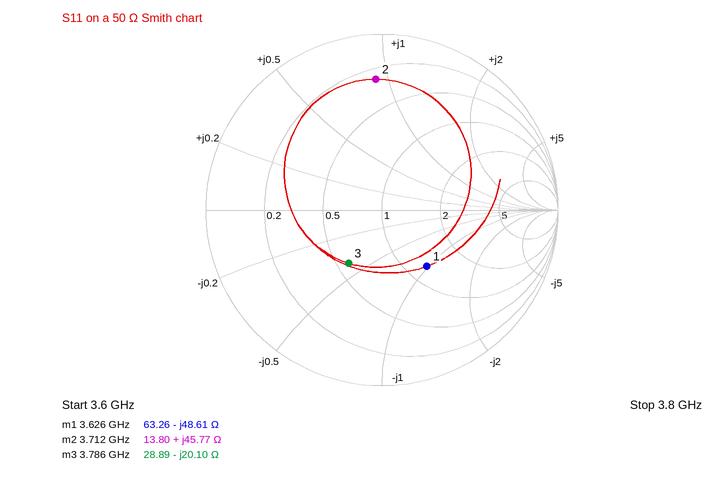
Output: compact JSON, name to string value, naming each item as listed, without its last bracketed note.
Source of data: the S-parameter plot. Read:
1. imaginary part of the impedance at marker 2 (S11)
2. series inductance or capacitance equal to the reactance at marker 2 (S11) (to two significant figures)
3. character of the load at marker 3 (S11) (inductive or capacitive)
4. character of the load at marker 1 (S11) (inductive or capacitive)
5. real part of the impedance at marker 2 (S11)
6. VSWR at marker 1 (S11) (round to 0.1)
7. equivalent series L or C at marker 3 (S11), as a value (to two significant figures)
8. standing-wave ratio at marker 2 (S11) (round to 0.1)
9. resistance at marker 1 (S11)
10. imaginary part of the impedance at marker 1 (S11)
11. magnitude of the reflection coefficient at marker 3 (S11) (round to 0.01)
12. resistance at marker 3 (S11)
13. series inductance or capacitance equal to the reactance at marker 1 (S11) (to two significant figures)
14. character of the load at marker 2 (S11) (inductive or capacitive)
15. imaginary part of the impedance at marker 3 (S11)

{"imaginary part of the impedance at marker 2": "+45.77 Ω", "series inductance or capacitance equal to the reactance at marker 2 (S11)": "2.0 nH", "character of the load at marker 3 (S11)": "capacitive", "character of the load at marker 1 (S11)": "capacitive", "real part of the impedance at marker 2": "13.80 Ω", "VSWR at marker 1 (S11)": "2.4", "equivalent series L or C at marker 3 (S11), as a value": "2.1 pF", "standing-wave ratio at marker 2 (S11)": "6.8", "resistance at marker 1": "63.26 Ω", "imaginary part of the impedance at marker 1": "-48.61 Ω", "magnitude of the reflection coefficient at marker 3 (S11)": "0.36", "resistance at marker 3": "28.89 Ω", "series inductance or capacitance equal to the reactance at marker 1 (S11)": "900 fF", "character of the load at marker 2 (S11)": "inductive", "imaginary part of the impedance at marker 3": "-20.10 Ω"}
